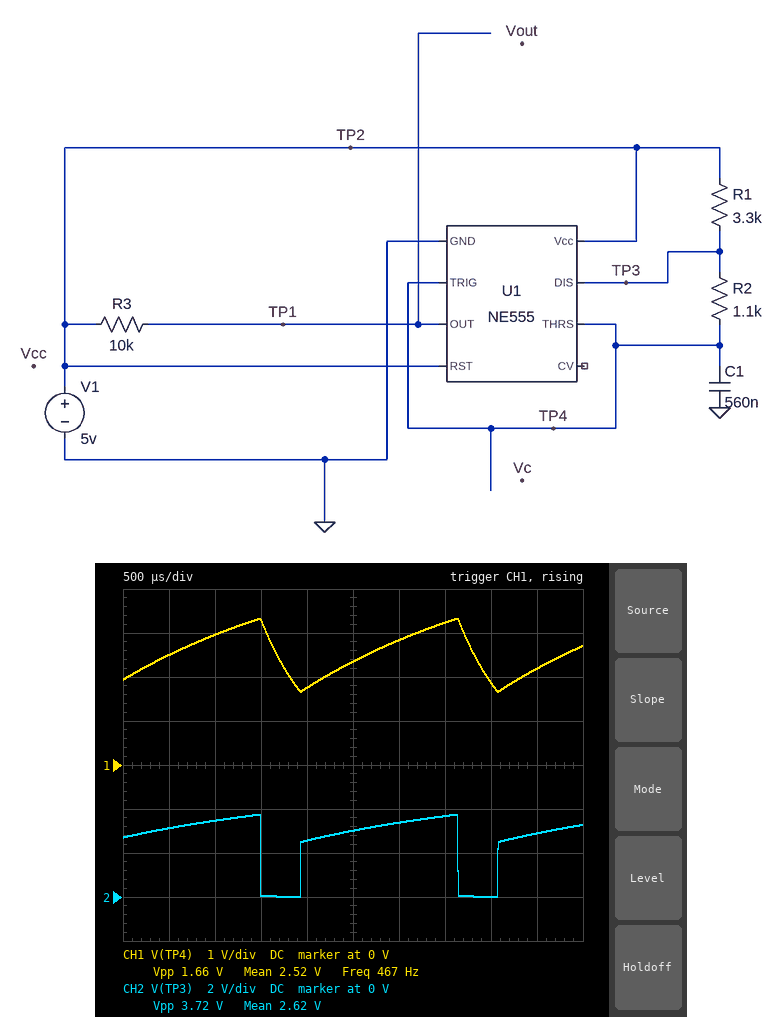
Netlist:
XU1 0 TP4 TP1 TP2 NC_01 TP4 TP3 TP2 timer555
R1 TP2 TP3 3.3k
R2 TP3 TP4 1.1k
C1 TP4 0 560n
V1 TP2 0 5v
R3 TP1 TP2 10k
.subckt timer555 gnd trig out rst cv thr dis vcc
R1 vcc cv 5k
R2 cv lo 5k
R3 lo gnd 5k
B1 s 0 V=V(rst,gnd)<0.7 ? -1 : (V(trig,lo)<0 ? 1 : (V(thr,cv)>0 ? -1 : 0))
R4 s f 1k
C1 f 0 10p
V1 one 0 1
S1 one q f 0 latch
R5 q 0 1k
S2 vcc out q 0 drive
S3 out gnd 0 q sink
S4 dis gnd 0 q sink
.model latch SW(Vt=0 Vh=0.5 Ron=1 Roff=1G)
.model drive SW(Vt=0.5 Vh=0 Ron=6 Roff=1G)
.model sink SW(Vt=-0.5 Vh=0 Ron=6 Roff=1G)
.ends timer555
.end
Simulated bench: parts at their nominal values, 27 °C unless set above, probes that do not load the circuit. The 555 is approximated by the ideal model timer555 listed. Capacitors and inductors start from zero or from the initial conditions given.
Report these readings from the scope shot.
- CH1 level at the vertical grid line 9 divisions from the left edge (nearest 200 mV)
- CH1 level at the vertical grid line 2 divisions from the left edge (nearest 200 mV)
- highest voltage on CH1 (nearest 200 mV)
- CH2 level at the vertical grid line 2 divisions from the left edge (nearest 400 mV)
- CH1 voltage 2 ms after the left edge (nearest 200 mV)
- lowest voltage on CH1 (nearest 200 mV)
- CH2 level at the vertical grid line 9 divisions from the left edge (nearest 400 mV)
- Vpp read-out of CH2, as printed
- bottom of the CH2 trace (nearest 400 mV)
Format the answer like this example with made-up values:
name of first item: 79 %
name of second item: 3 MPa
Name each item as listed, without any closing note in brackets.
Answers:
CH1 level at the vertical grid line 9 divisions from the left edge: 2.2 V
CH1 level at the vertical grid line 2 divisions from the left edge: 3.0 V
highest voltage on CH1: 3.4 V
CH2 level at the vertical grid line 2 divisions from the left edge: 3.6 V
CH1 voltage 2 ms after the left edge: 1.8 V
lowest voltage on CH1: 1.6 V
CH2 level at the vertical grid line 9 divisions from the left edge: 2.8 V
Vpp read-out of CH2, as printed: 3.72 V
bottom of the CH2 trace: 0 V
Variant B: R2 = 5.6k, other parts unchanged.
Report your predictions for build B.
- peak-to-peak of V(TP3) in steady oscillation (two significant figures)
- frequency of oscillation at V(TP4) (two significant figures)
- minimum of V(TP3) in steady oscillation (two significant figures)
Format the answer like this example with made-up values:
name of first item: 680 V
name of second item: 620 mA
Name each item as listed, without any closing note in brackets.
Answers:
peak-to-peak of V(TP3) in steady oscillation: 4.4 V
frequency of oscillation at V(TP4): 180 Hz
minimum of V(TP3) in steady oscillation: 11 mV
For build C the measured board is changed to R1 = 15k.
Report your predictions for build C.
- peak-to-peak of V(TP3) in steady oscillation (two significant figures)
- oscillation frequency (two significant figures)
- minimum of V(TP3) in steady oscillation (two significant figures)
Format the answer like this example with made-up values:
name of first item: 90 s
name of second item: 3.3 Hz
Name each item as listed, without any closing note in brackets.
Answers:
peak-to-peak of V(TP3) in steady oscillation: 3.4 V
oscillation frequency: 150 Hz
minimum of V(TP3) in steady oscillation: 11 mV
